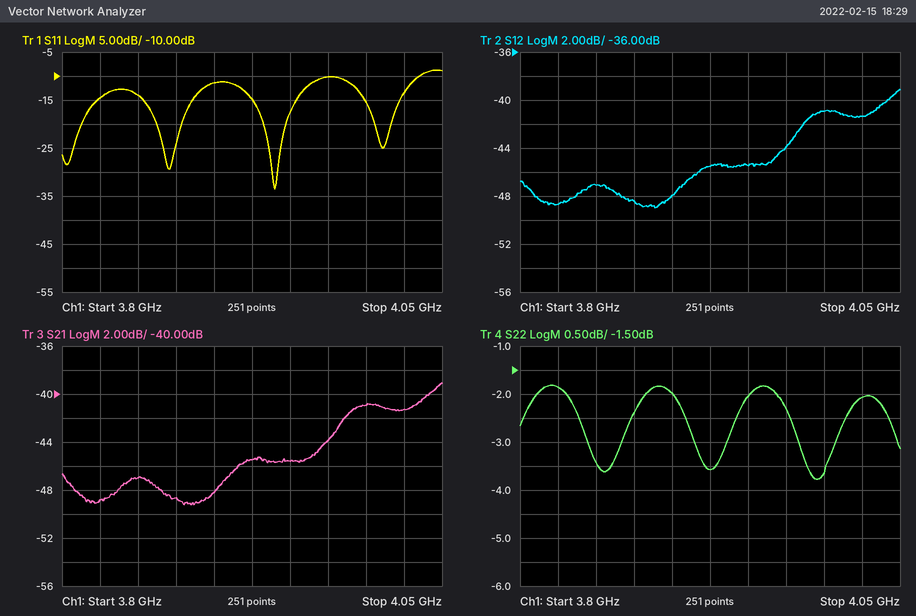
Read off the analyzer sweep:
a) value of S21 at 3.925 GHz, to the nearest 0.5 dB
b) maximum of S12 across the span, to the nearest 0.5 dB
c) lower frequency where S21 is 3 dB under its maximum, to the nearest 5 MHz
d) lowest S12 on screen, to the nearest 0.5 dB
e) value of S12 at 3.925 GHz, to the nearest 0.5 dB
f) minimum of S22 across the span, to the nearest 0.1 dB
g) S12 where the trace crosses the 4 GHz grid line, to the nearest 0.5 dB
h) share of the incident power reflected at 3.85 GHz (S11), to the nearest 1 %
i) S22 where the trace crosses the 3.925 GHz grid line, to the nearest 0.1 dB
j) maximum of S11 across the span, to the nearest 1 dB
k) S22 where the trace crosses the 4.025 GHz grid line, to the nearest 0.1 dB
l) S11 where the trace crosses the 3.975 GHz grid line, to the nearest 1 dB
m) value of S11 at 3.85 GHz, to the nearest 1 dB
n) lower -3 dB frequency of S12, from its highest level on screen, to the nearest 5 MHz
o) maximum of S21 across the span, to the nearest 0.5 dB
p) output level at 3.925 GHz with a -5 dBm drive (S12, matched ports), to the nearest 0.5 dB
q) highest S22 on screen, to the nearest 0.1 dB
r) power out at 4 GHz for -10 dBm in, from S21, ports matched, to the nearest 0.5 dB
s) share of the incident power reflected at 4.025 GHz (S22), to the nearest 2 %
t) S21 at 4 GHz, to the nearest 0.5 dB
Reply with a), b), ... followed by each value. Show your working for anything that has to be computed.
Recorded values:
a) -45.5 dB
b) -39.0 dB
c) 3.985 GHz
d) -49.0 dB
e) -45.5 dB
f) -3.8 dB
g) -41.0 dB
h) 10^(-14/10) ≈ 4 %
i) -3.6 dB
j) -9 dB
k) -2.1 dB
l) -10 dB
m) -14 dB
n) 3.985 GHz
o) -39.0 dB
p) -5 dBm + (-45.5 dB) = -50.5 dBm
q) -1.8 dB
r) -10 dBm + (-41.0 dB) = -51.0 dBm
s) 10^(-2.1/10) ≈ 62 %
t) -41.0 dB
